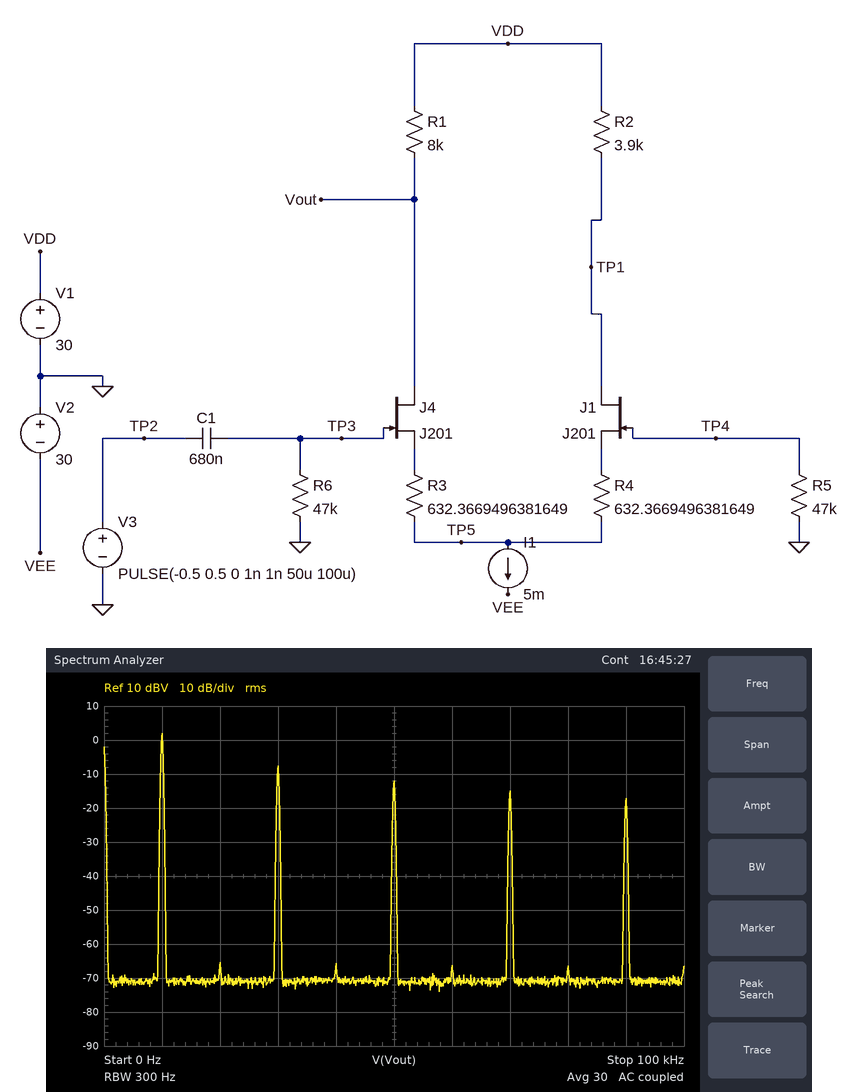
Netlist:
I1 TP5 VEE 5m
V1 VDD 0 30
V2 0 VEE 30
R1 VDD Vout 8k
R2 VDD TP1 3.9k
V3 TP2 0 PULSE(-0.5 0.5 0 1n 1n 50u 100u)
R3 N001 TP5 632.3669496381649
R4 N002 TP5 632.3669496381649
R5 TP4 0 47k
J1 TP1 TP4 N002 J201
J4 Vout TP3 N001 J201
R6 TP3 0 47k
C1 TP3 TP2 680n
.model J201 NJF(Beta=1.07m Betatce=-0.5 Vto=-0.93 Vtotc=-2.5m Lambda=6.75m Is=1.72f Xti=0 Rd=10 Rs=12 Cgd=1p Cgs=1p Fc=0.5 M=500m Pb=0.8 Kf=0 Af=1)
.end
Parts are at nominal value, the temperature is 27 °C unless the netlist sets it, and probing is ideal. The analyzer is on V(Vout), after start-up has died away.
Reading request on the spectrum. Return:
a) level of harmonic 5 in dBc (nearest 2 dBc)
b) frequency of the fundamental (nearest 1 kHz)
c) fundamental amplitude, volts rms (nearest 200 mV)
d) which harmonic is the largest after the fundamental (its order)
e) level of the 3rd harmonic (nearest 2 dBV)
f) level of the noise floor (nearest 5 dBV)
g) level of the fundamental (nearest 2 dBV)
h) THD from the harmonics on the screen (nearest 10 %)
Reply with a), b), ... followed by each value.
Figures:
a) -14 dBc
b) 10 kHz
c) 1.2 V
d) 3
e) -8 dBV
f) -70 dBV
g) 2 dBV
h) 40 %
